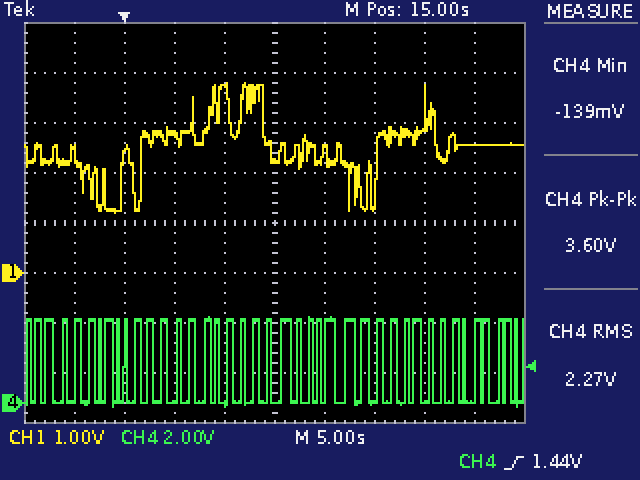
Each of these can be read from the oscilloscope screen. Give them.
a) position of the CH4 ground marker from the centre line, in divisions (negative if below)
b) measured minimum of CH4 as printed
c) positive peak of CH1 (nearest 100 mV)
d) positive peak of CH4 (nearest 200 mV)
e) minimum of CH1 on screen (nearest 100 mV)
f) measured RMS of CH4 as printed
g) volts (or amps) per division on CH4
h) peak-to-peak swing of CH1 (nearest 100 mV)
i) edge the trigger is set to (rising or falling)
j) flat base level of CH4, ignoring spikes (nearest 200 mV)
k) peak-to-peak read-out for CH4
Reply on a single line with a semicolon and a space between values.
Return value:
-3.6 div; -139 mV; 3.8 V; 3.4 V; 1.2 V; 2.27 V; 2 V; 2.6 V; rising; 0.0 V; 3.60 V
